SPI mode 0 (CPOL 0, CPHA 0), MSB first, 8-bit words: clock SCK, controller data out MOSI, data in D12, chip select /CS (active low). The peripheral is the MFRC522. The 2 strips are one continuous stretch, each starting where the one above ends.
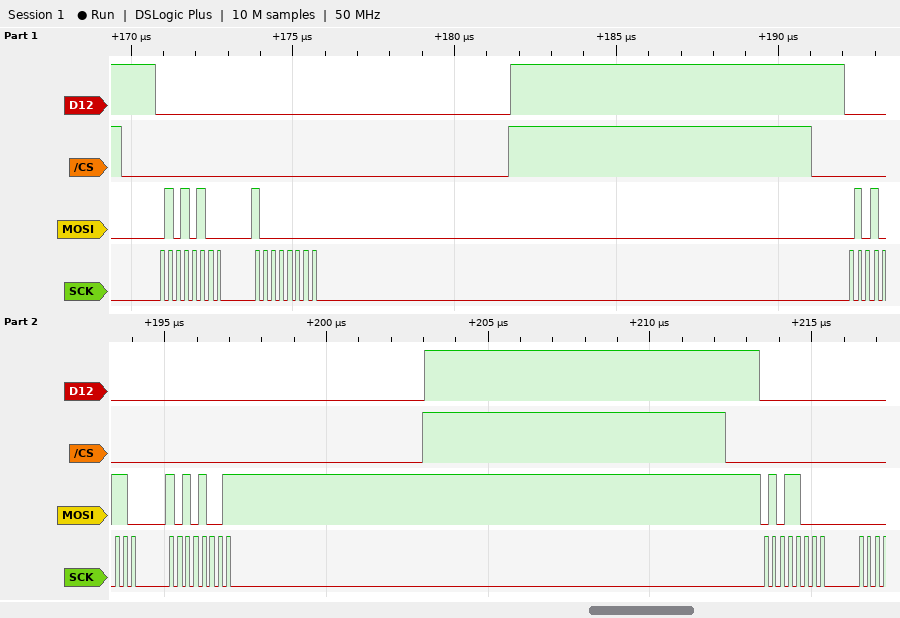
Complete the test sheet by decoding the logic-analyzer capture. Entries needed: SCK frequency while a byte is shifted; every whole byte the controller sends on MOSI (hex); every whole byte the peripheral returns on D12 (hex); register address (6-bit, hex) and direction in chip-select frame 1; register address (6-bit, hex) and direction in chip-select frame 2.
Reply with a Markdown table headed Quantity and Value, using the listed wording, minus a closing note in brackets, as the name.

| Quantity | Value |
|---|---|
| SCK frequency while a byte is shifted | 4 MHz |
| every whole byte the controller sends on MOSI | 0x54 0x80 0x56 0xA9 0x58 |
| every whole byte the peripheral returns on D12 | 0x00 0x00 0x00 0x00 0x00 |
| register address (6-bit, hex) and direction in chip-select frame 1 | 0x2A write |
| register address (6-bit, hex) and direction in chip-select frame 2 | 0x2B write |
